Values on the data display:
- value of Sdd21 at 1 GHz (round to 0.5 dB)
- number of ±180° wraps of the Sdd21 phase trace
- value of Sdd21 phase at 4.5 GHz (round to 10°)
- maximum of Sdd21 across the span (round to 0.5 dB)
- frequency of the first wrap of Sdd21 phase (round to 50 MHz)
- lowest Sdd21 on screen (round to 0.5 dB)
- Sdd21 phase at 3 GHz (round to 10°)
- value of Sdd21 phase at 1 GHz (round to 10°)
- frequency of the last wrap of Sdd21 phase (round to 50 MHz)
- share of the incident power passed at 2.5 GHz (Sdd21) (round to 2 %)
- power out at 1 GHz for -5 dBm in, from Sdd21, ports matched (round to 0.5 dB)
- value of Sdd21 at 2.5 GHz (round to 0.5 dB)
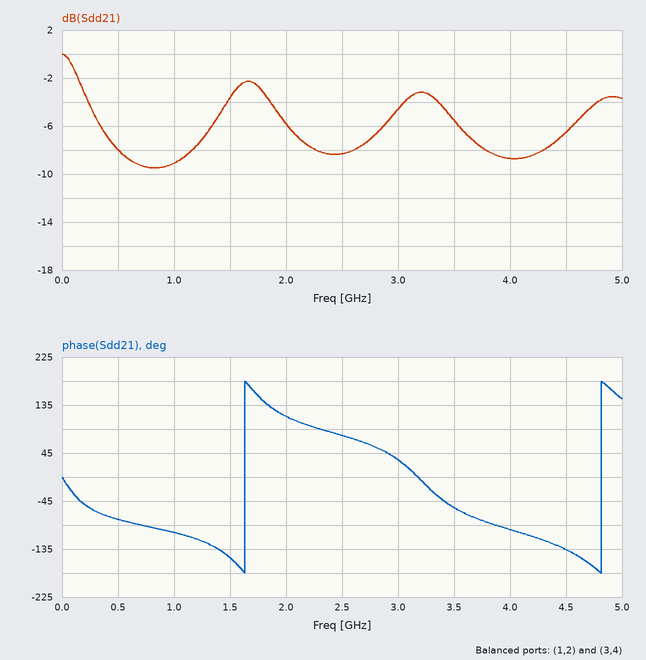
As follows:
-9.0 dB
2
-140°
0.0 dB
1.65 GHz
-9.5 dB
30°
-100°
4.80 GHz
14 %
-14.0 dBm
-8.5 dB
